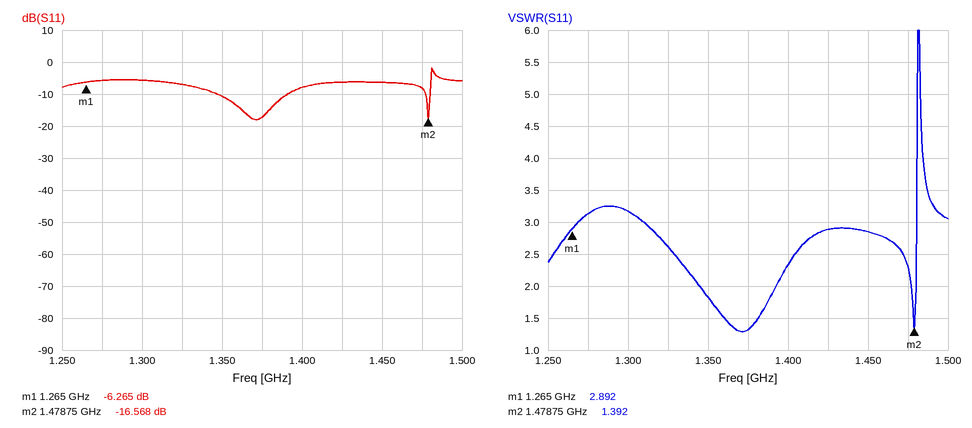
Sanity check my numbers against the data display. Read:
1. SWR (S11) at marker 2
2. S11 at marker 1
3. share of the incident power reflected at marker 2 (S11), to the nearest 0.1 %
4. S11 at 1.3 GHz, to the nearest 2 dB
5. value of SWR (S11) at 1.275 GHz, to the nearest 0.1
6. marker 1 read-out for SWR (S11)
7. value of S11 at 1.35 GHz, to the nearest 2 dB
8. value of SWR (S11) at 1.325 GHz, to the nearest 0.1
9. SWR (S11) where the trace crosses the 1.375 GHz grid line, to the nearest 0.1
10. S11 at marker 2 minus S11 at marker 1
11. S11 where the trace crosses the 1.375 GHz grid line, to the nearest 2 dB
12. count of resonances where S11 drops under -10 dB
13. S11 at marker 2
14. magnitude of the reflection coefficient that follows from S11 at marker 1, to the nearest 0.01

1.392
-6.265 dB
2.2 %
-6 dB
3.1
2.892
-10 dB
2.6
1.3
-10.303 dB
-18 dB
2
-16.568 dB
0.49
